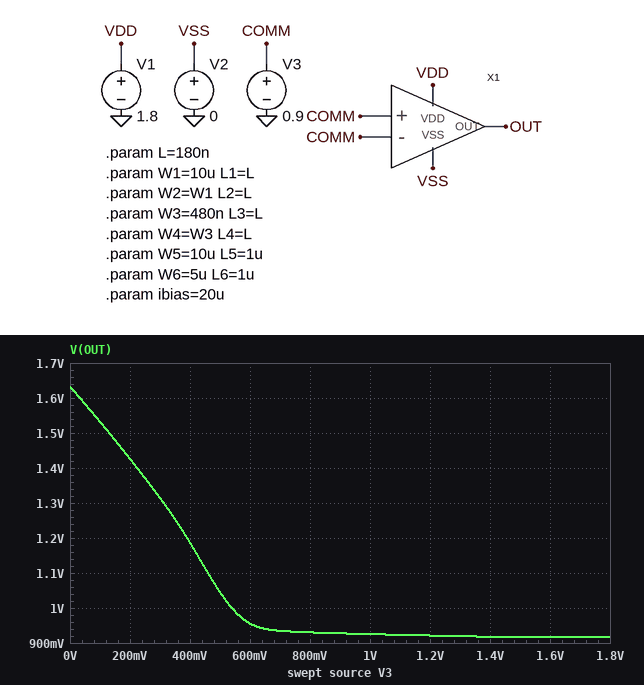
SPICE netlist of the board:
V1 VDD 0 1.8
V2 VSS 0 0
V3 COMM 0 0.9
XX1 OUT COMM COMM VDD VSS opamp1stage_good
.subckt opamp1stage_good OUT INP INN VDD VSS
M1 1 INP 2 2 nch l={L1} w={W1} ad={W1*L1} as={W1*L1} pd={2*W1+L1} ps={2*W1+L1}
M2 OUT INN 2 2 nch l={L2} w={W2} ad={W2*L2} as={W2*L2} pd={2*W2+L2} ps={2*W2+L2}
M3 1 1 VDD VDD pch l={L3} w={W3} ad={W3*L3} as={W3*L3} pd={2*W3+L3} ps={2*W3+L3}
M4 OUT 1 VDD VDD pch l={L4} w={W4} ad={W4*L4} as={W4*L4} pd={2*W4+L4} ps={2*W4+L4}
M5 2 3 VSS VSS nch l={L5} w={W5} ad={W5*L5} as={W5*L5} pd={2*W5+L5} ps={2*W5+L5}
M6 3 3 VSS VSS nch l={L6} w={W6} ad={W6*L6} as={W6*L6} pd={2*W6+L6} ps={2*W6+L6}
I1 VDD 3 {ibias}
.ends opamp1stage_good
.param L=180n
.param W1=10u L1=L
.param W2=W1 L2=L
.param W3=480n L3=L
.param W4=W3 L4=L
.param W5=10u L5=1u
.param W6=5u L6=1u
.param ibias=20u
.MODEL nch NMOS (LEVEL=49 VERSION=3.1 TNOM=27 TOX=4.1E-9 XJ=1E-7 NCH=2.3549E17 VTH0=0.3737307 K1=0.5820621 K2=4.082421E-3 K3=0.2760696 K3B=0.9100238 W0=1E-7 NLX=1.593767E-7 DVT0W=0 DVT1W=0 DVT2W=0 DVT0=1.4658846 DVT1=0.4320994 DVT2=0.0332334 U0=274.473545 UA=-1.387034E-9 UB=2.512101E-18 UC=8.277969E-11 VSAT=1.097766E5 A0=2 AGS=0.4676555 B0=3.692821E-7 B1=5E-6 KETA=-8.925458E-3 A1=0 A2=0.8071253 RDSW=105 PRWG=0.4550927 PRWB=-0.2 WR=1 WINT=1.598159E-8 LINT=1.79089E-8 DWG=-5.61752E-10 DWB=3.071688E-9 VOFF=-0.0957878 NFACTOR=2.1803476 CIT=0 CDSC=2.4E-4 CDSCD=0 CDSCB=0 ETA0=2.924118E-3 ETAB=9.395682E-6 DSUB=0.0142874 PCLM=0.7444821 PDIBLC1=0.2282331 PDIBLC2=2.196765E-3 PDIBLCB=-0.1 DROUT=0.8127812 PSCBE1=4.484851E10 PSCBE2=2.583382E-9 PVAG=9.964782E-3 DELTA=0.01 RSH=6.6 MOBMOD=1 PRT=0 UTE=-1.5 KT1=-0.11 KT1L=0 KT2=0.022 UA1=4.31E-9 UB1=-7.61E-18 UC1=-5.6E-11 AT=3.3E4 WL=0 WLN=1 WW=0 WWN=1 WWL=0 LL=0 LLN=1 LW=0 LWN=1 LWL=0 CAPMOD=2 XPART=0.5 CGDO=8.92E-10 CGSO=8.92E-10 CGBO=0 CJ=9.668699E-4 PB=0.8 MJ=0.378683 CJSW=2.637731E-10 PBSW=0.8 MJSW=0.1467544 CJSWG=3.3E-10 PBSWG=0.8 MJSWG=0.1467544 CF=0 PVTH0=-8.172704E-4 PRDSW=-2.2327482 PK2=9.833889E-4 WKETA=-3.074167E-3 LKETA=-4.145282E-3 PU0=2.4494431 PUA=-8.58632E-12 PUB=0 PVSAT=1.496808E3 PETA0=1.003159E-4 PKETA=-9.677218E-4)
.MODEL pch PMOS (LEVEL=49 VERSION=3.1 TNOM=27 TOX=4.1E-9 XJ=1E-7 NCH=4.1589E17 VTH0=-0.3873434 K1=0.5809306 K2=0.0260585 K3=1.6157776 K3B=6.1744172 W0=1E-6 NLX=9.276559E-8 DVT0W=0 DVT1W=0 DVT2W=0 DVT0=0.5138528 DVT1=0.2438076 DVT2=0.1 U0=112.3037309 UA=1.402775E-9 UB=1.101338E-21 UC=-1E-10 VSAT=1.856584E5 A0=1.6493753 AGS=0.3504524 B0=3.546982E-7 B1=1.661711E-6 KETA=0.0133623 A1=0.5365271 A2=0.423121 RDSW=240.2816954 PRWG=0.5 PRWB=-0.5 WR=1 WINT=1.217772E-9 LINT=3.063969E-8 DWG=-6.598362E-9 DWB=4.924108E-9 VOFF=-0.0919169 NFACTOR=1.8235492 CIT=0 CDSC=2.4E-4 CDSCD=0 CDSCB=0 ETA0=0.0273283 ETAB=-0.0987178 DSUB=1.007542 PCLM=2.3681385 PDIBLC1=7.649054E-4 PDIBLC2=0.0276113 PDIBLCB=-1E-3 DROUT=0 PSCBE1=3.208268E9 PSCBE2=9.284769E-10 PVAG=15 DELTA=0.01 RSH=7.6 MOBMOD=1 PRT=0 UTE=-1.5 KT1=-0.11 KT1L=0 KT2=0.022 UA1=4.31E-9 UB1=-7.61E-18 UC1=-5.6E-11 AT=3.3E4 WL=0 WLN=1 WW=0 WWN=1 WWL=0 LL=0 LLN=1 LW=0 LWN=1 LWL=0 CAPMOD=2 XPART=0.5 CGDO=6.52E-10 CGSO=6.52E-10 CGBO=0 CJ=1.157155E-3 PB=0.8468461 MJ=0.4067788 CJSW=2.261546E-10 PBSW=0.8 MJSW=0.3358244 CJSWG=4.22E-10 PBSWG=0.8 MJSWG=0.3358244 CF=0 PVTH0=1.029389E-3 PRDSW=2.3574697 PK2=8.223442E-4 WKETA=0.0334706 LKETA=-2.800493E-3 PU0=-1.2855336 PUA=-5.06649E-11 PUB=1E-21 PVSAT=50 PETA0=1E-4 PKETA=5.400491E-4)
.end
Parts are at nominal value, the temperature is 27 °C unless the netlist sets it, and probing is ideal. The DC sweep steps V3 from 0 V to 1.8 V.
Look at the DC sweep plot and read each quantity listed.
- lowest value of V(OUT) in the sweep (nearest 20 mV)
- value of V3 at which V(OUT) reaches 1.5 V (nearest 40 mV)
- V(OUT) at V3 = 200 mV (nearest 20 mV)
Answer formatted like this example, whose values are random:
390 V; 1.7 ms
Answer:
920 mV; 120 mV; 1.42 V
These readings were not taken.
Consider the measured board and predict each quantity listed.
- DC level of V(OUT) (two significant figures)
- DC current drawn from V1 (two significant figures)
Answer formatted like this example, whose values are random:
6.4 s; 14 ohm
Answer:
930 mV; 59 µA
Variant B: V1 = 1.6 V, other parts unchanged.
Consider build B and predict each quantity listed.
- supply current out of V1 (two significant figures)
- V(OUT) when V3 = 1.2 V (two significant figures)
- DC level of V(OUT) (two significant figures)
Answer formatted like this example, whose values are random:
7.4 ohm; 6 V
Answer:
59 µA; 720 mV; 730 mV
